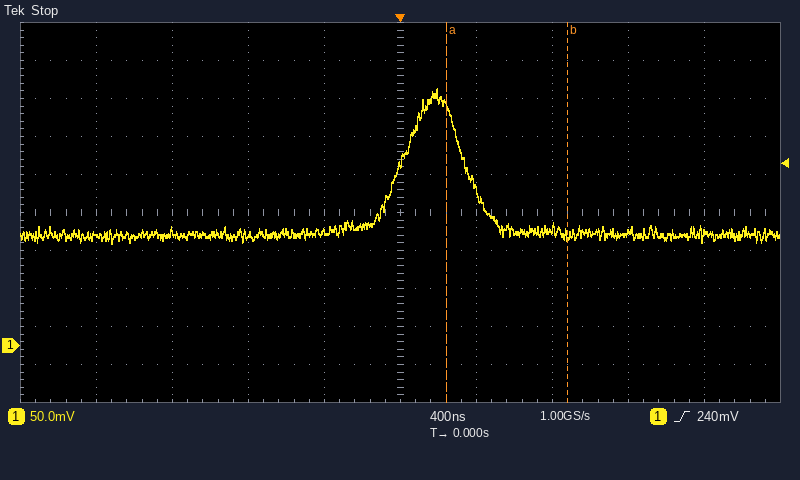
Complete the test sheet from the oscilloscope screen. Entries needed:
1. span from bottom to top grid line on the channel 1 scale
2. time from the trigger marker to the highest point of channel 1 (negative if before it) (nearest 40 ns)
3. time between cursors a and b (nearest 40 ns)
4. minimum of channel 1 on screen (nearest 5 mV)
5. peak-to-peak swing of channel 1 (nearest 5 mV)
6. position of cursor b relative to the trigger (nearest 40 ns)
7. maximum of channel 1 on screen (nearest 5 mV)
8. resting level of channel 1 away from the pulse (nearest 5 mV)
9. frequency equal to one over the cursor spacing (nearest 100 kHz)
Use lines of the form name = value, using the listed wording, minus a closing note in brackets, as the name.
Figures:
span from bottom to top grid line on the channel 1 scale = 500 mV
time from the trigger marker to the highest point of channel 1 (negative if before it) = +200 ns
time between cursors a and b = 640 ns
minimum of channel 1 on screen = 135 mV
peak-to-peak swing of channel 1 = 205 mV
position of cursor b relative to the trigger = +880 ns
maximum of channel 1 on screen = 340 mV
resting level of channel 1 away from the pulse = 145 mV
frequency equal to one over the cursor spacing = 1.6 MHz
